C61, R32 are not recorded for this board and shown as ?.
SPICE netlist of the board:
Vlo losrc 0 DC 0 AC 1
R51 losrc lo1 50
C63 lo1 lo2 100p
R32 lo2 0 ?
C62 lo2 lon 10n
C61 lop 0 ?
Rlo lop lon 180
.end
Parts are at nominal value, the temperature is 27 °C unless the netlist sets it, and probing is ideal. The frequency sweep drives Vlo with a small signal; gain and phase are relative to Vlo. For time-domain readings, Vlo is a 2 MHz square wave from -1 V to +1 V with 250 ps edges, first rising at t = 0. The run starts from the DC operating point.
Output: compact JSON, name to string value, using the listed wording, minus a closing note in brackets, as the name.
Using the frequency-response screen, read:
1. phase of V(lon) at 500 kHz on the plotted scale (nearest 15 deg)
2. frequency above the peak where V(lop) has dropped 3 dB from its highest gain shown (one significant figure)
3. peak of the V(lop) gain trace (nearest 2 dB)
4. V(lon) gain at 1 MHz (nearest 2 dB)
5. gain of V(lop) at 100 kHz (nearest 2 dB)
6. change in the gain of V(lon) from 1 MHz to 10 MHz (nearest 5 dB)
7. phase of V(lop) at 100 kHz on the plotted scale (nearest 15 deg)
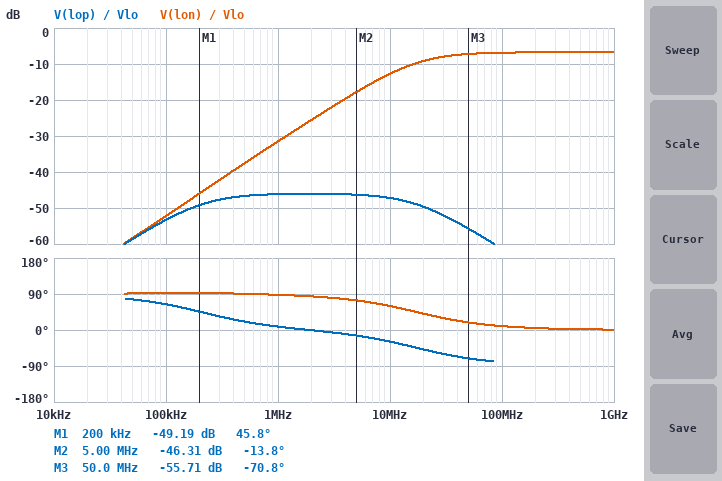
{"phase of V(lon) at 500 kHz on the plotted scale": "90 deg", "frequency above the peak where V(lop) has dropped 3 dB from its highest gain shown": "20 MHz", "peak of the V(lop) gain trace": "-46 dB", "V(lon) gain at 1 MHz": "-32 dB", "gain of V(lop) at 100 kHz": "-54 dB", "change in the gain of V(lon) from 1 MHz to 10 MHz": "20 dB", "phase of V(lop) at 100 kHz on the plotted scale": "60 deg"}
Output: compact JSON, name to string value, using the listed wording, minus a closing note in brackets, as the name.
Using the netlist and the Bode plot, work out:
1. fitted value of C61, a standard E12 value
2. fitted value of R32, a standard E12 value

{"fitted value of C61, a standard E12 value": "4.7 nF", "fitted value of R32, a standard E12 value": "56 Ω"}
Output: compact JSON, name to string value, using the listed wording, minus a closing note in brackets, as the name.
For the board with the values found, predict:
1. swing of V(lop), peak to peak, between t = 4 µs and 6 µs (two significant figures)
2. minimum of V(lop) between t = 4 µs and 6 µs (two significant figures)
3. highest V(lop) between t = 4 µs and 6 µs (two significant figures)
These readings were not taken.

{"swing of V(lop), peak to peak, between t = 4 µs and 6 µs": "11 mV", "minimum of V(lop) between t = 4 µs and 6 µs": "-5.5 mV", "highest V(lop) between t = 4 µs and 6 µs": "5.5 mV"}
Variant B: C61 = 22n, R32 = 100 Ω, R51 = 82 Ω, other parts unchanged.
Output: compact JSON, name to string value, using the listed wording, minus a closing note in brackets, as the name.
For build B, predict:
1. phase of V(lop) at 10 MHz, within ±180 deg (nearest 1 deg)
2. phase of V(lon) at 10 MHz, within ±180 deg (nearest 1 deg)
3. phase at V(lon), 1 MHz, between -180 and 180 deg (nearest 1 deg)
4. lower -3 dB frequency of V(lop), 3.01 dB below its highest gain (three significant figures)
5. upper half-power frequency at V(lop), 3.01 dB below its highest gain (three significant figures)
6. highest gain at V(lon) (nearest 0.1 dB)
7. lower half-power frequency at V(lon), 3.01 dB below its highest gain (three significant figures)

{"phase of V(lop) at 10 MHz, within ±180 deg": "-42 deg", "phase of V(lon) at 10 MHz, within ±180 deg": "48 deg", "phase at V(lon), 1 MHz, between -180 and 180 deg": "87 deg", "lower -3 dB frequency of V(lop), 3.01 dB below its highest gain": "81.3 kHz", "upper half-power frequency at V(lop), 3.01 dB below its highest gain": "11.1 MHz", "highest gain at V(lon)": "-7.1 dB", "lower half-power frequency at V(lon), 3.01 dB below its highest gain": "10.9 MHz"}
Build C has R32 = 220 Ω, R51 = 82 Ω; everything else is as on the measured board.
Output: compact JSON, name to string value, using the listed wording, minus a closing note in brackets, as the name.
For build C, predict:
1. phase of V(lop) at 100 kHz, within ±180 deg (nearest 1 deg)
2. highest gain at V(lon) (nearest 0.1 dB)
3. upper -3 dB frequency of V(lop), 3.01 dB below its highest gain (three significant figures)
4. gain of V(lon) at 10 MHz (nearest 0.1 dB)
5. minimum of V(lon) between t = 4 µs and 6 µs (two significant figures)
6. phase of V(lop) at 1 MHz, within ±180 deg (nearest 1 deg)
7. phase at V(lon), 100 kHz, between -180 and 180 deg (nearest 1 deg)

{"phase of V(lop) at 100 kHz, within ±180 deg": "50 deg", "highest gain at V(lon)": "-5.2 dB", "upper -3 dB frequency of V(lop), 3.01 dB below its highest gain": "9.12 MHz", "gain of V(lon) at 10 MHz": "-7.8 dB", "minimum of V(lon) between t = 4 µs and 6 µs": "-1.1 V", "phase of V(lop) at 1 MHz, within ±180 deg": "1 deg", "phase at V(lon), 100 kHz, between -180 and 180 deg": "78 deg"}
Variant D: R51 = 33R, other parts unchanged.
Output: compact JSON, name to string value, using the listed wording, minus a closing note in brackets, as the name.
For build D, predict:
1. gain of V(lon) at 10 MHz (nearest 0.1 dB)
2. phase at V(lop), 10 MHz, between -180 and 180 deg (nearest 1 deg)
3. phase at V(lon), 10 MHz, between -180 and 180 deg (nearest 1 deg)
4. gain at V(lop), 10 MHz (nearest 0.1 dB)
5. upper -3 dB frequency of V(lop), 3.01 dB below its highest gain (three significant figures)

{"gain of V(lon) at 10 MHz": "-12.3 dB", "phase at V(lop), 10 MHz, between -180 and 180 deg": "-24 deg", "phase at V(lon), 10 MHz, between -180 and 180 deg": "65 deg", "gain at V(lop), 10 MHz": "-46.8 dB", "upper -3 dB frequency of V(lop), 3.01 dB below its highest gain": "21.5 MHz"}
